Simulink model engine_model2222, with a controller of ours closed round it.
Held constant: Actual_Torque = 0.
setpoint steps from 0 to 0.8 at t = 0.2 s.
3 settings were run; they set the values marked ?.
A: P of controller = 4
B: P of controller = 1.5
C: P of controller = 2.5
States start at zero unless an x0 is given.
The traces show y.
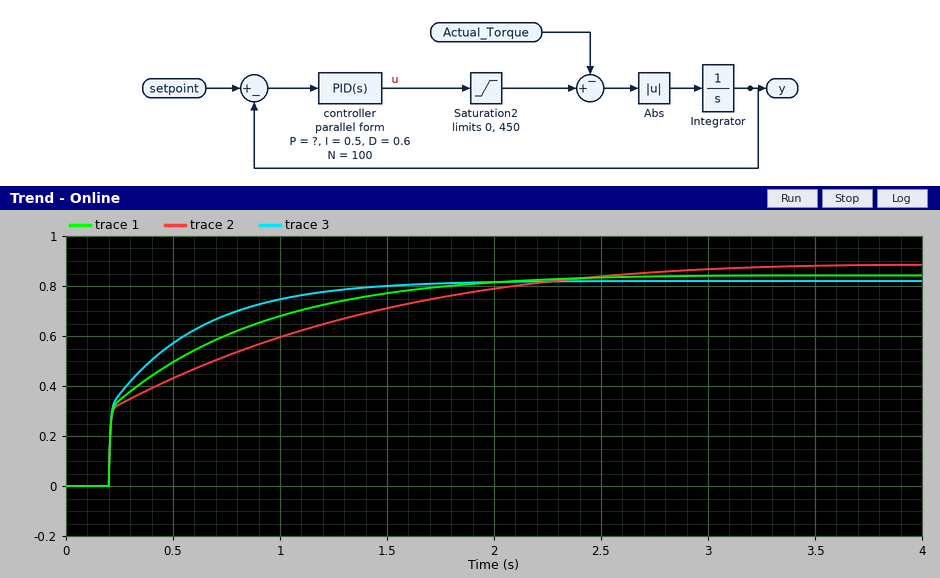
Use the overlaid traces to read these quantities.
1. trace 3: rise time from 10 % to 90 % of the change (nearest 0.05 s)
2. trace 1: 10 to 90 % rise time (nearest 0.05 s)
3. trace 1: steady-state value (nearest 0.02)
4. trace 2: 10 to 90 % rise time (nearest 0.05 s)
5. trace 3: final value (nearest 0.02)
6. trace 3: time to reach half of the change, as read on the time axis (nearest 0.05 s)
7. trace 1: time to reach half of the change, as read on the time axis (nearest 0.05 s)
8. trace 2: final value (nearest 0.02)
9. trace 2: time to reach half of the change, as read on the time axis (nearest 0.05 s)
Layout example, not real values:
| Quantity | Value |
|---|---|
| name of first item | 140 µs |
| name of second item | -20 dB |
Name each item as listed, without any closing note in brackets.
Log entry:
| Quantity | Value |
|---|---|
| trace 3: rise time from 10 % to 90 % of the change | 0.75 s |
| trace 1: 10 to 90 % rise time | 1.20 s |
| trace 1: steady-state value | 0.84 |
| trace 2: 10 to 90 % rise time | 1.85 s |
| trace 3: final value | 0.82 |
| trace 3: time to reach half of the change, as read on the time axis | 0.30 s |
| trace 1: time to reach half of the change, as read on the time axis | 0.35 s |
| trace 2: final value | 0.88 |
| trace 2: time to reach half of the change, as read on the time axis | 0.55 s |
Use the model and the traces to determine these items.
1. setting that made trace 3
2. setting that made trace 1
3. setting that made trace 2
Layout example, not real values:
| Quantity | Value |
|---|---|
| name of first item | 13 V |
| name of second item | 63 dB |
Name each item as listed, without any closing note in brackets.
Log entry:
| Quantity | Value |
|---|---|
| setting that made trace 3 | A |
| setting that made trace 1 | C |
| setting that made trace 2 | B |
